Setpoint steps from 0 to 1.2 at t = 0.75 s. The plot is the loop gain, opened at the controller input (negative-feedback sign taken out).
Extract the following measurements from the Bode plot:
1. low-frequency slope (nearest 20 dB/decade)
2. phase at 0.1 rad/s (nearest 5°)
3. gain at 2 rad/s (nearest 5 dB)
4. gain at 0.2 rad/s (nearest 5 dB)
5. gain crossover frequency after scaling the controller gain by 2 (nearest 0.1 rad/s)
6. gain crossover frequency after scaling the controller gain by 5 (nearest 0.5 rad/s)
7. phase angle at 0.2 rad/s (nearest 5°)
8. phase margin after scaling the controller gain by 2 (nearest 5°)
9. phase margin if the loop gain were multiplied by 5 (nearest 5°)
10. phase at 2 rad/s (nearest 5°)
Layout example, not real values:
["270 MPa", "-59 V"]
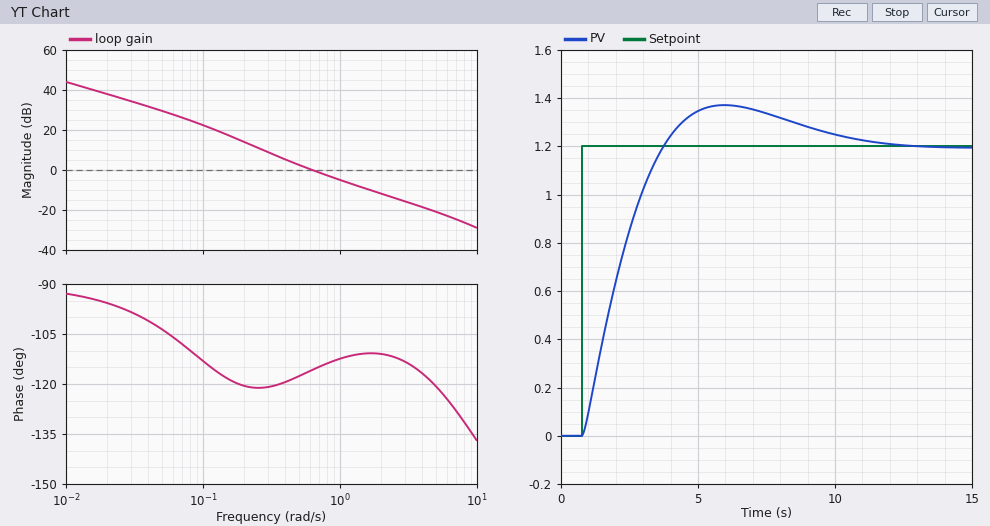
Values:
["-20 dB/decade", "-115°", "-10 dB", "15 dB", "1.1 rad/s", "2.5 rad/s", "-120°", "70°", "70°", "-110°"]
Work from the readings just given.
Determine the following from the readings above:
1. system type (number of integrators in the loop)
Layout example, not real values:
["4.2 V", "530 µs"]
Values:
["1"]
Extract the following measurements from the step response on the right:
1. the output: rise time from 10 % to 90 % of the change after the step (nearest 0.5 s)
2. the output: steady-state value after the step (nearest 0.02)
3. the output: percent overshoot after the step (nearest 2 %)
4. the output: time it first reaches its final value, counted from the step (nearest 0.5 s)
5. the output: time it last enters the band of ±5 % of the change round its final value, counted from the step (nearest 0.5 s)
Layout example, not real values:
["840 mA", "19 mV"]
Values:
["2.0 s", "1.20", "14 %", "3.0 s", "9.0 s"]
